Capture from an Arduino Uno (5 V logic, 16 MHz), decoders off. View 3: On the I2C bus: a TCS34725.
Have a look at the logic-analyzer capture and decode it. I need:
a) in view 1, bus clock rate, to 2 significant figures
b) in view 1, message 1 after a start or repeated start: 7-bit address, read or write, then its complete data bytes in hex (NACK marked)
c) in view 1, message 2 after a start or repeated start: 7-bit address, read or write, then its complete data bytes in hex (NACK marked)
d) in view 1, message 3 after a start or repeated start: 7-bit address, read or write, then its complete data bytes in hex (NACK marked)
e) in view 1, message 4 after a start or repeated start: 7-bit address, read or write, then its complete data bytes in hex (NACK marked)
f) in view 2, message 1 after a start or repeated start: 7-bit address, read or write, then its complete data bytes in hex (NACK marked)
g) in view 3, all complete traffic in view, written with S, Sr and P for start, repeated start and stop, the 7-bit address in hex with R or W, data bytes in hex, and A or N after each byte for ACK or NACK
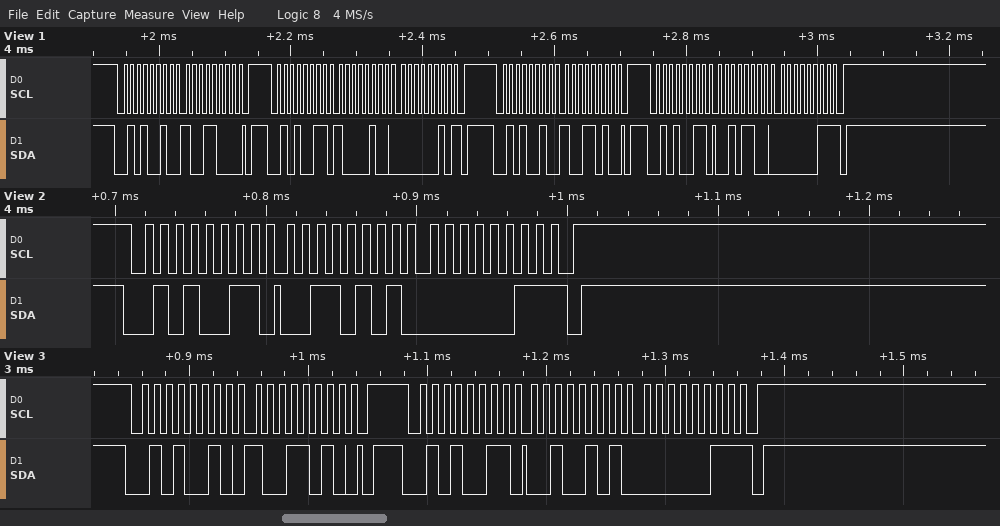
100 kHz
0x29 write: 98
0x29 read: 84 02 NACK
0x29 write: 9A
0x29 read: 2C 03 NACK
0x29 read: 35 03 NACK
S 29W A 9A A P S 29R A 25 A 03 N P
